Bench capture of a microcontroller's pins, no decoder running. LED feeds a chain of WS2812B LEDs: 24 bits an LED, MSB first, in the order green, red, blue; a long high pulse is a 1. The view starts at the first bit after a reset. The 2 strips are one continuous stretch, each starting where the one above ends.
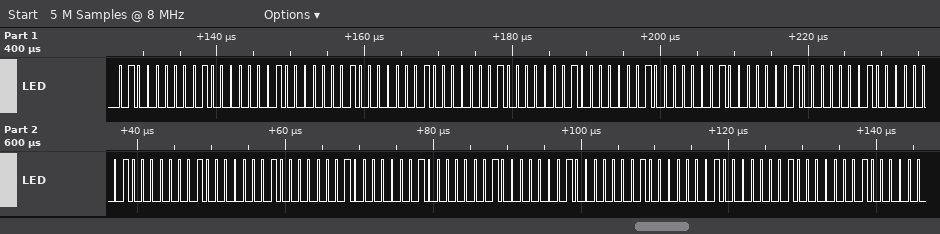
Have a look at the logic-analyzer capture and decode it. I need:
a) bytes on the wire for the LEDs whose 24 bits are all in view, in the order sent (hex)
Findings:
40 40 40 40 40 40 40 40 40 40 40 40 40 40 40 40 40 40 40 40 40
